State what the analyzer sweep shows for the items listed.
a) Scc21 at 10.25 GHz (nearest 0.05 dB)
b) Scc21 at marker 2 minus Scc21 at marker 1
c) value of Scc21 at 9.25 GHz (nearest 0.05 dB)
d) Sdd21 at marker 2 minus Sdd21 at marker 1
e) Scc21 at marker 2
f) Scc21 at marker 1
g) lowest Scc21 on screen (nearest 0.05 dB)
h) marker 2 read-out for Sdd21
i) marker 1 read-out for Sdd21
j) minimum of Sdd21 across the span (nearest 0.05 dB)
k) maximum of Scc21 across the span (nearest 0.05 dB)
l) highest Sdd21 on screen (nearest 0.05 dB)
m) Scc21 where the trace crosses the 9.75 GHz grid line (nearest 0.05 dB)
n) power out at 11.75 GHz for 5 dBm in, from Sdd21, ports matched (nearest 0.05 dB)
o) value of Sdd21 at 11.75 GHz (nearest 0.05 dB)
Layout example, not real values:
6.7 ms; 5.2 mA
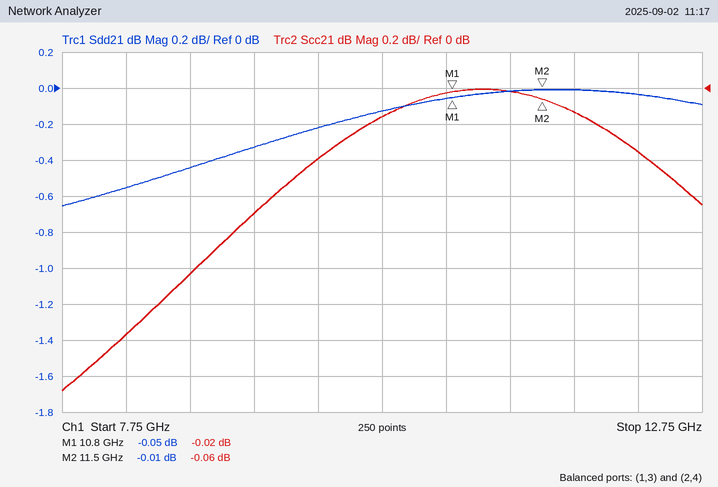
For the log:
-0.15 dB; -0.04 dB; -0.70 dB; 0.04 dB; -0.06 dB; -0.02 dB; -1.70 dB; -0.01 dB; -0.05 dB; -0.65 dB; 0.00 dB; 0.00 dB; -0.40 dB; 5.00 dBm; 0.00 dB
